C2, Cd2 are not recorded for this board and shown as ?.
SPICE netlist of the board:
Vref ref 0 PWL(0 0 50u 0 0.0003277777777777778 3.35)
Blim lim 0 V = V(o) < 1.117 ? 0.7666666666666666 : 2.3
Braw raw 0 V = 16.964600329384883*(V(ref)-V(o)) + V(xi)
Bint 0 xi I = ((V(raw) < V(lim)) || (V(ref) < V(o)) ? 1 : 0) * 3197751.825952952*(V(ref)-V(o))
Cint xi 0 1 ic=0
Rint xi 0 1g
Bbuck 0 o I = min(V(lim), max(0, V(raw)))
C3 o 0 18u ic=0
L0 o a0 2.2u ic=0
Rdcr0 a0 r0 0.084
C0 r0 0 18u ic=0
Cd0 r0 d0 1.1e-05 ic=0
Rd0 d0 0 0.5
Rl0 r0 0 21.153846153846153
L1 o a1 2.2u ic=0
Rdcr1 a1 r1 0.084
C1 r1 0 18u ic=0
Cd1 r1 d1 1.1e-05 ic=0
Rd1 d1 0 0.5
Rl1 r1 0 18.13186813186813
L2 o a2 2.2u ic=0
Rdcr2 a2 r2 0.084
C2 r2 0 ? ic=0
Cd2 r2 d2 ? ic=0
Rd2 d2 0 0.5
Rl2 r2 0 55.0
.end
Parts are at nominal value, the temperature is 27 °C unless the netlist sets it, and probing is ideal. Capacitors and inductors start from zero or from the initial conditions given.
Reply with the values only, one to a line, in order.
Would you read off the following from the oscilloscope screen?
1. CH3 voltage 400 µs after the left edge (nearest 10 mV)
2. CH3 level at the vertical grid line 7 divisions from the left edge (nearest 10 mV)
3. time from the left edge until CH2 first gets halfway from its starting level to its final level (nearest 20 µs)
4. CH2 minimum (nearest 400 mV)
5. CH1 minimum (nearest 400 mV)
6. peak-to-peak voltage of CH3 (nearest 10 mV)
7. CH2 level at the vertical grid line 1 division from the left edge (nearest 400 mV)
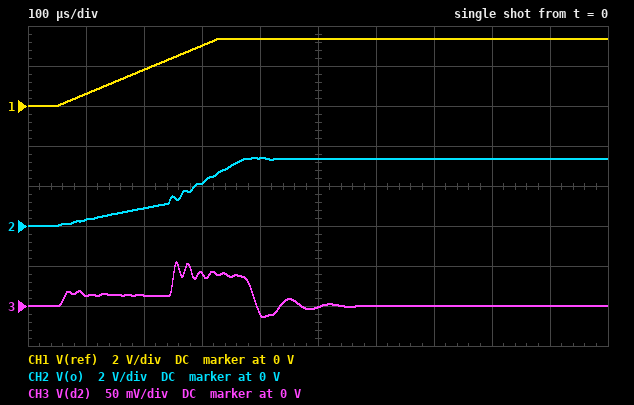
-10 mV
0 V
260 µs
0 V
0 V
70 mV
400 mV
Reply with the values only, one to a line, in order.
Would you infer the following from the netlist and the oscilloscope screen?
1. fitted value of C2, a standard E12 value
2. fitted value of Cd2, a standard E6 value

39 µF
4.7 µF
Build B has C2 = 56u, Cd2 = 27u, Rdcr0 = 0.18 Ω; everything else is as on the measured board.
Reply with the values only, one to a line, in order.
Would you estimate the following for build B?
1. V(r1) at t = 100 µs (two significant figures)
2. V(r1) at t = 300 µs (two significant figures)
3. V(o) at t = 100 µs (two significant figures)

230 mV
1.1 V
250 mV
